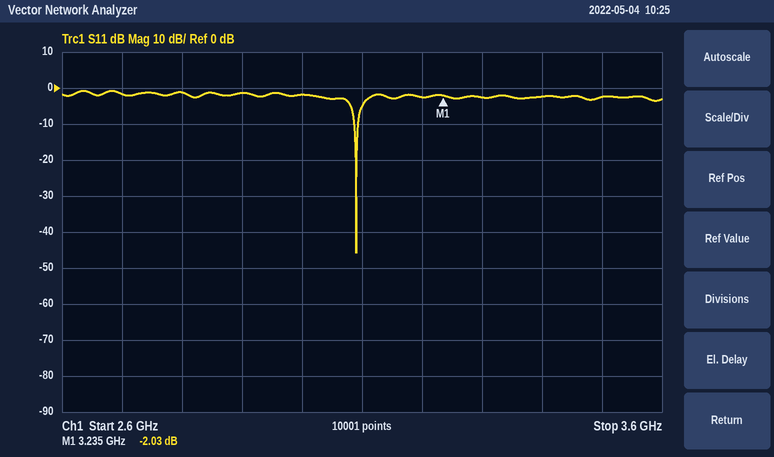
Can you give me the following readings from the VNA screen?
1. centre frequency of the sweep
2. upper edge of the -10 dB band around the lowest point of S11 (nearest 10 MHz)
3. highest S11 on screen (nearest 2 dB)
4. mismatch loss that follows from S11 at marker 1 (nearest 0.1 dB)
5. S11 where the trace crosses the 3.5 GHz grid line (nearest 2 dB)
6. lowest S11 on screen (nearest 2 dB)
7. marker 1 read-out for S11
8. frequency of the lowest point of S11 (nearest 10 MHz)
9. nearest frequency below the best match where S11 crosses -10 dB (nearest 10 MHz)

3.1 GHz
3.09 GHz
0 dB
4.3 dB
-2 dB
-46 dB
-2.03 dB
3.09 GHz
3.09 GHz
